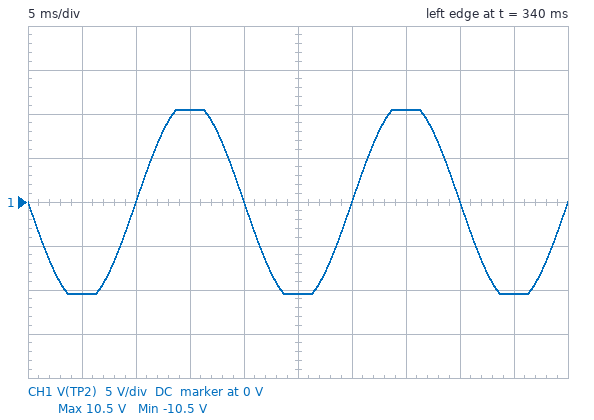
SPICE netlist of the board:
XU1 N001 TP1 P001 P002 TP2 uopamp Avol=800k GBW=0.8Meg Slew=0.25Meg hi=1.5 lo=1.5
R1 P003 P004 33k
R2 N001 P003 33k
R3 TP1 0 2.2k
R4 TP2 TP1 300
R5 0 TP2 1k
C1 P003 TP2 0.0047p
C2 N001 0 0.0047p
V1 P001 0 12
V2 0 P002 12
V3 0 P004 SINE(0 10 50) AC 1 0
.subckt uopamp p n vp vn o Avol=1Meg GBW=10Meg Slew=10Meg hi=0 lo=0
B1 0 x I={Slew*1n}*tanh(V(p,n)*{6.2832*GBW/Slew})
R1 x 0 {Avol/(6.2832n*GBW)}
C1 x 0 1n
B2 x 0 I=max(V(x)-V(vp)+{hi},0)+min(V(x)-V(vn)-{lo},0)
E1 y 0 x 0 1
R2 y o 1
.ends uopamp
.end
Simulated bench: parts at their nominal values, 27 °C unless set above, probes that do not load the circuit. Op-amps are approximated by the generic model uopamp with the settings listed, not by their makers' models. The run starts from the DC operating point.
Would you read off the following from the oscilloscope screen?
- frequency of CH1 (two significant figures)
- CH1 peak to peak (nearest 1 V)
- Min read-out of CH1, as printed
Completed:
50 Hz
21 V
-10.5 V
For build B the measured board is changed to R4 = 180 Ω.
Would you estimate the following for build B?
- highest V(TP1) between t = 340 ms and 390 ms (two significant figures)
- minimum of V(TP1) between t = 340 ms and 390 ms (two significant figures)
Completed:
9.7 V
-9.7 V
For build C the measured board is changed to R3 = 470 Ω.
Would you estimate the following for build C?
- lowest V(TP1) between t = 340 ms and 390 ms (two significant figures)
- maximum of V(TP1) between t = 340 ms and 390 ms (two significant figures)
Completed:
-6.4 V
6.4 V
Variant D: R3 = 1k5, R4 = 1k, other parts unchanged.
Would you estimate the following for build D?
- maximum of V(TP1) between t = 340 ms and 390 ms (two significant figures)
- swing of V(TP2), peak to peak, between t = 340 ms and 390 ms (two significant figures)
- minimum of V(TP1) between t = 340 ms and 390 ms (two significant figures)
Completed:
6.3 V
21 V
-6.3 V
